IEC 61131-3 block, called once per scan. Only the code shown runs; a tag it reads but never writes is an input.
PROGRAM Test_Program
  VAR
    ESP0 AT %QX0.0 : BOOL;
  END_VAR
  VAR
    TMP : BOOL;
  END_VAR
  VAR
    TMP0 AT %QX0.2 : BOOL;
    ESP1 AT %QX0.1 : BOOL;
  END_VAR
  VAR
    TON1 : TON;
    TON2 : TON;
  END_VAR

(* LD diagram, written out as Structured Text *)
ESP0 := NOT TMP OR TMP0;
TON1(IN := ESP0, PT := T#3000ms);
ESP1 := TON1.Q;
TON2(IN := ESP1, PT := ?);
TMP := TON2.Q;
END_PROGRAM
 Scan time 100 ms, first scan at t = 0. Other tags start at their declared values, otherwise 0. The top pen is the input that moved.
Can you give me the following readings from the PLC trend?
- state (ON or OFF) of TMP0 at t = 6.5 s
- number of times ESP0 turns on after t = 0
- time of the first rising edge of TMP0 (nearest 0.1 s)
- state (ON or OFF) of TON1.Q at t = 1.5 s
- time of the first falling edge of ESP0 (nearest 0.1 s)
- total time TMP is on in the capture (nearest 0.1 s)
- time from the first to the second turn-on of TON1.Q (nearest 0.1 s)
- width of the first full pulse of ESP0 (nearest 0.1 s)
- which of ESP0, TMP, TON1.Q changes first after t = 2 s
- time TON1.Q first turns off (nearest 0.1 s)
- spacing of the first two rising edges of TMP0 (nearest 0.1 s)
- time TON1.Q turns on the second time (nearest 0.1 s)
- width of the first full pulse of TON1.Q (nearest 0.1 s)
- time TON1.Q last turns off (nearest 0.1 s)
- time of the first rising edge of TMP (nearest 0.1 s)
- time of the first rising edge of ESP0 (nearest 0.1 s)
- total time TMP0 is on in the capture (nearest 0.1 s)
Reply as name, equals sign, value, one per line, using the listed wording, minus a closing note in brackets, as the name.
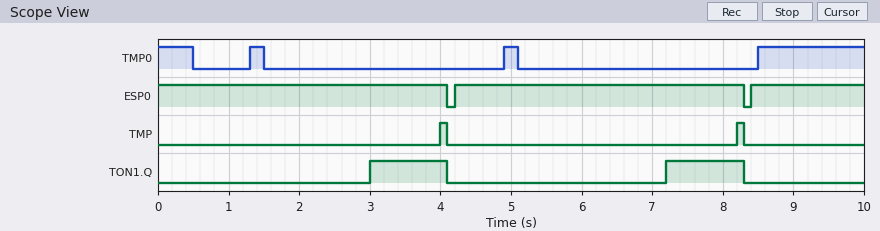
state (ON or OFF) of TMP0 at t = 6.5 s = OFF
number of times ESP0 turns on after t = 0 = 2
time of the first rising edge of TMP0 = 1.3 s
state (ON or OFF) of TON1.Q at t = 1.5 s = OFF
time of the first falling edge of ESP0 = 4.1 s
total time TMP is on in the capture = 0.2 s
time from the first to the second turn-on of TON1.Q = 4.2 s
width of the first full pulse of ESP0 = 4.1 s
which of ESP0, TMP, TON1.Q changes first after t = 2 s = TON1.Q
time TON1.Q first turns off = 4.1 s
spacing of the first two rising edges of TMP0 = 3.6 s
time TON1.Q turns on the second time = 7.2 s
width of the first full pulse of TON1.Q = 1.1 s
time TON1.Q last turns off = 8.3 s
time of the first rising edge of TMP = 4.0 s
time of the first rising edge of ESP0 = 4.2 s
total time TMP0 is on in the capture = 2.4 s
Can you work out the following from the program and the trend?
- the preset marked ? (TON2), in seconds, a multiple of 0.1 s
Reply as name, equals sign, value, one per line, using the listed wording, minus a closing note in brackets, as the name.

the preset marked ? (TON2), in seconds, a multiple of 0.1 s = 1.0 s
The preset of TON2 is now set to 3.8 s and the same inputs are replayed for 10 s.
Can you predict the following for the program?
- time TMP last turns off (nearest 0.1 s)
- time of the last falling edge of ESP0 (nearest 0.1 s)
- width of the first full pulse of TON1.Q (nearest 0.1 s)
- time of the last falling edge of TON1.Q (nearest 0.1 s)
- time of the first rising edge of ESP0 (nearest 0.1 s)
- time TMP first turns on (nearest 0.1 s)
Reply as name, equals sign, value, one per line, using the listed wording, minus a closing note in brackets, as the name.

time TMP last turns off = 6.9 s
time of the last falling edge of ESP0 = 6.9 s
width of the first full pulse of TON1.Q = 3.9 s
time of the last falling edge of TON1.Q = 6.9 s
time of the first rising edge of ESP0 = 7.0 s
time TMP first turns on = 6.8 s
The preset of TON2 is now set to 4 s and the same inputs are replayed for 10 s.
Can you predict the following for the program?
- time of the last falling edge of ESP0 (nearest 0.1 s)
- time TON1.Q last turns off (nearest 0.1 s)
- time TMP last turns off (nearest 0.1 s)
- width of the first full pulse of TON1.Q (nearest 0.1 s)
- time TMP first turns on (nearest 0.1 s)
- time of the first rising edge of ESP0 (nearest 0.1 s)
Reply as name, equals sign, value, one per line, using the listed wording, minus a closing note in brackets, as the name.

time of the last falling edge of ESP0 = 7.1 s
time TON1.Q last turns off = 7.1 s
time TMP last turns off = 7.1 s
width of the first full pulse of TON1.Q = 4.1 s
time TMP first turns on = 7.0 s
time of the first rising edge of ESP0 = 7.2 s
